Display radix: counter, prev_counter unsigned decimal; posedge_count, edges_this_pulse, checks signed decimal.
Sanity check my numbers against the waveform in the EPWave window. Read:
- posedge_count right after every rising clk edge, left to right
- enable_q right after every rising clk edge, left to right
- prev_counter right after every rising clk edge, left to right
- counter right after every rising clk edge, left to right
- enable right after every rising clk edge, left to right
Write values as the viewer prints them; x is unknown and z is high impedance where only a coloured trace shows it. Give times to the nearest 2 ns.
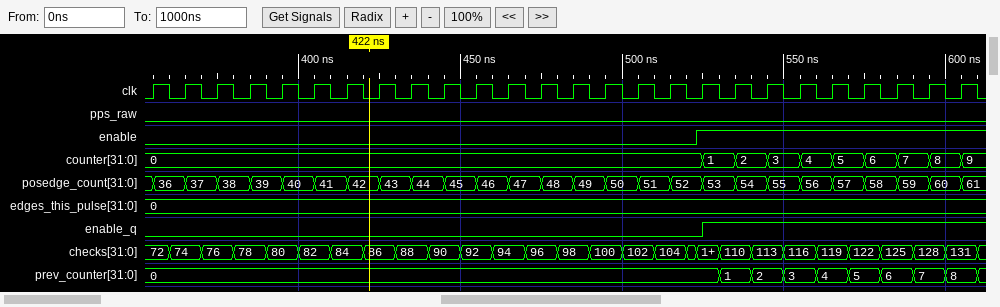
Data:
36, 37, 38, 39, 40, 41, 42, 43, 44, 45, 46, 47, 48, 49, 50, 51, 52, 53, 54, 55, 56, 57, 58, 59, 60, 61
0 0 0 0 0 0 0 0 0 0 0 0 0 0 0 0 0 1 1 1 1 1 1 1 1 1
0, 0, 0, 0, 0, 0, 0, 0, 0, 0, 0, 0, 0, 0, 0, 0, 0, 0, 1, 2, 3, 4, 5, 6, 7, 8
0, 0, 0, 0, 0, 0, 0, 0, 0, 0, 0, 0, 0, 0, 0, 0, 0, 1, 2, 3, 4, 5, 6, 7, 8, 9
0 0 0 0 0 0 0 0 0 0 0 0 0 0 0 0 0 1 1 1 1 1 1 1 1 1
